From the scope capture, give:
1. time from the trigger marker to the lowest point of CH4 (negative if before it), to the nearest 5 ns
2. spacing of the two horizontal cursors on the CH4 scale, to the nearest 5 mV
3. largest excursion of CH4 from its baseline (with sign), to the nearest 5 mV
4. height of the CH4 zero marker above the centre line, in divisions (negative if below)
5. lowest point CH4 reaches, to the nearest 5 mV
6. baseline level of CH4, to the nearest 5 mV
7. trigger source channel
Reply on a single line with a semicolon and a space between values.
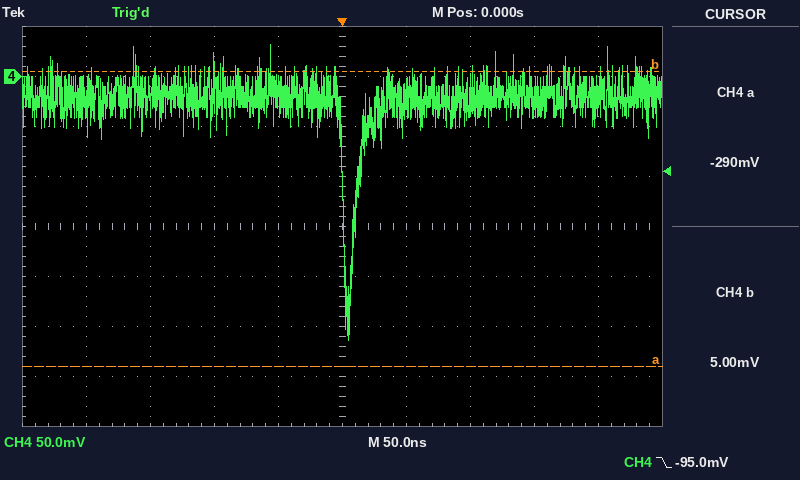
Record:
+5 ns; 295 mV; -245 mV; +3.0 div; -265 mV; -20 mV; CH4
